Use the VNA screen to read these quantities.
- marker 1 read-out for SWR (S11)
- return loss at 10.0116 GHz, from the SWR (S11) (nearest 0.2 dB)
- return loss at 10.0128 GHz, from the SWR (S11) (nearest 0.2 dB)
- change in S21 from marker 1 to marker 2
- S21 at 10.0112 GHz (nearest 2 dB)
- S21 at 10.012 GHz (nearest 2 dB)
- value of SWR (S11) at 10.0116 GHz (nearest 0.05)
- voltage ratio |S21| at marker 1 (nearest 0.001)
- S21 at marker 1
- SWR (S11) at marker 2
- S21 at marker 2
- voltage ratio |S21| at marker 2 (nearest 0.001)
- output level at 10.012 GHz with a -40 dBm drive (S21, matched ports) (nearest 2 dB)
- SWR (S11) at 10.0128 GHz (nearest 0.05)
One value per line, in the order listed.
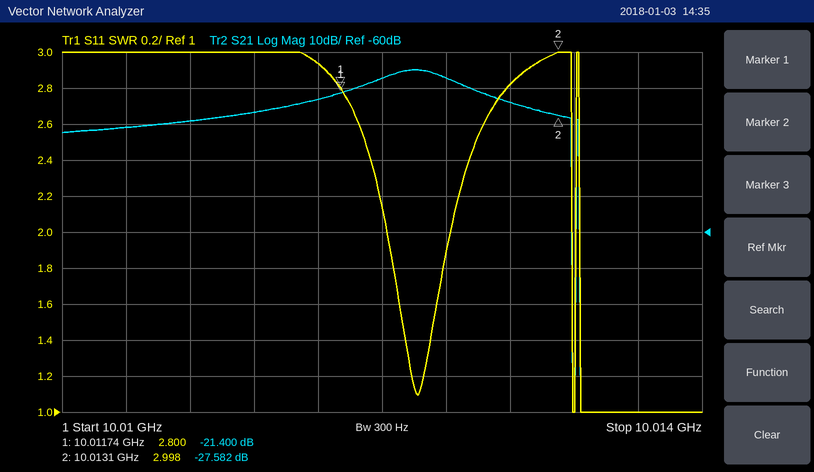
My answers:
2.800
6.2 dB
6.4 dB
-6.182 dB
-26 dB
-18 dB
2.95
0.085
-21.400 dB
2.998
-27.582 dB
0.042
-58 dBm
2.80
